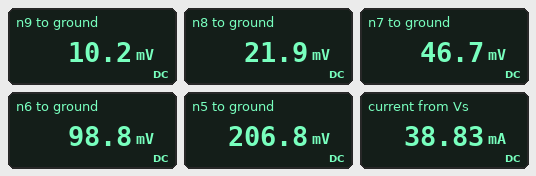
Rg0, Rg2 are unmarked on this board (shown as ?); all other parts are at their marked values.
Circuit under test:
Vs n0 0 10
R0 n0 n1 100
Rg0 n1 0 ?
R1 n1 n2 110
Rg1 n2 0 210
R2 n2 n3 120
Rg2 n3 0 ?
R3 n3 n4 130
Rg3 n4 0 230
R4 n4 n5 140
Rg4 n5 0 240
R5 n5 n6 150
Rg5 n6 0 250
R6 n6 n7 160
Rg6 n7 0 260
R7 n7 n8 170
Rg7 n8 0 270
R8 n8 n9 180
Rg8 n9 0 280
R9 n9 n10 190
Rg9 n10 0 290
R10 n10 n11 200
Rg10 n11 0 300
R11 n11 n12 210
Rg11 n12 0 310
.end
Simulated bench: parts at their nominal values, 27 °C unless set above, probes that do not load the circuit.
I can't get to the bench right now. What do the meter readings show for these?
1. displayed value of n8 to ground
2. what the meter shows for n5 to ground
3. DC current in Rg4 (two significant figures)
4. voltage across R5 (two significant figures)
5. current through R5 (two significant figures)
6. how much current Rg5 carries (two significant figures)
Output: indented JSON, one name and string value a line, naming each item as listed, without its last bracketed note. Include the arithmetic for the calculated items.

{
  "displayed value of n8 to ground": "21.9 mV",
  "what the meter shows for n5 to ground": "206.8 mV",
  "DC current in Rg4": "(206.8 mV) / 240 Ω = 860 µA",
  "voltage across R5": "206.8 mV - 98.8 mV = 110 mV",
  "current through R5": "(206.8 mV - 98.8 mV) / 150 Ω = 720 µA",
  "how much current Rg5 carries": "(98.8 mV) / 250 Ω = 400 µA"
}
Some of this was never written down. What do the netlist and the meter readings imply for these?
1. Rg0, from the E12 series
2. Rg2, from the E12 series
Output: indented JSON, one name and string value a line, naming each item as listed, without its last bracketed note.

{
  "Rg0, from the E12 series": "680 Ω",
  "Rg2, from the E12 series": "68 Ω"
}
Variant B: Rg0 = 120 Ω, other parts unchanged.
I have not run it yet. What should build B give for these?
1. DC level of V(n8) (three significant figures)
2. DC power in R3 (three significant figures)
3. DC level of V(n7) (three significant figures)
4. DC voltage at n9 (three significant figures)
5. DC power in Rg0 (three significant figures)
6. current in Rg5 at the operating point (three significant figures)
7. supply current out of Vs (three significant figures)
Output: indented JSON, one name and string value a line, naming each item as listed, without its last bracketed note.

{
  "DC level of V(n8)": "15.4 mV",
  "DC power in R3": "765 µW",
  "DC level of V(n7)": "32.9 mV",
  "DC voltage at n9": "7.17 mV",
  "DC power in Rg0": "155 mW",
  "current in Rg5 at the operating point": "278 µA",
  "supply current out of Vs": "56.9 mA"
}
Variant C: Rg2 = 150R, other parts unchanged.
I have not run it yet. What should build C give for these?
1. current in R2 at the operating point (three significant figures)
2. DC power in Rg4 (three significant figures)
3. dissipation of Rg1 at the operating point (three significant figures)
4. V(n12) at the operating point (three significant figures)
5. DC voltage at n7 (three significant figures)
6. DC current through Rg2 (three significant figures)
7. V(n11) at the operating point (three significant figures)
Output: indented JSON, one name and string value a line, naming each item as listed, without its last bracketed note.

{
  "current in R2 at the operating point": "14.2 mA",
  "DC power in Rg4": "418 µW",
  "dissipation of Rg1 at the operating point": "44.3 mW",
  "V(n12) at the operating point": "2.12 mV",
  "DC voltage at n7": "71.5 mV",
  "DC current through Rg2": "8.95 mA",
  "V(n11) at the operating point": "3.55 mV"
}
